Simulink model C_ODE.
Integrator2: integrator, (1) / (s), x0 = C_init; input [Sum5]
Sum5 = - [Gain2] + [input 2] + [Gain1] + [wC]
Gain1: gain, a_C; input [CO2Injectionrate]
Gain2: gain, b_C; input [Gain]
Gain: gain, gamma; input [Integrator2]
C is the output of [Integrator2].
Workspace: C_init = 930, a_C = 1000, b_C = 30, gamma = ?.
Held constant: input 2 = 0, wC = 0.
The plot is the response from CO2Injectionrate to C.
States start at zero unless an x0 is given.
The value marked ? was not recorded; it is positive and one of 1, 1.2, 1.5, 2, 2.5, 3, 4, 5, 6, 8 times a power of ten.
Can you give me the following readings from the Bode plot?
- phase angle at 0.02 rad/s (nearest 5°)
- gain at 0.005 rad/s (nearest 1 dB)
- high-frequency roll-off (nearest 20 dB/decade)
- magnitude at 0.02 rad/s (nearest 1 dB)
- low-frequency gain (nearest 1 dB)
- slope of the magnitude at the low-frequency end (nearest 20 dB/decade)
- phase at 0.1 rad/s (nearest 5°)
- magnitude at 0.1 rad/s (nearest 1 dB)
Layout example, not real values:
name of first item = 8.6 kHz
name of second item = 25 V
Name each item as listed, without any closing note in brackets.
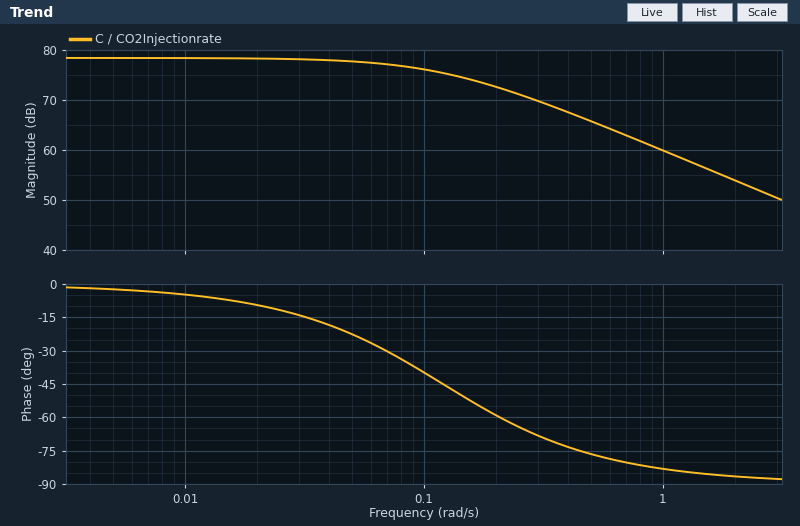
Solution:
phase angle at 0.02 rad/s = -10°
gain at 0.005 rad/s = 78 dB
high-frequency roll-off = -20 dB/decade
magnitude at 0.02 rad/s = 78 dB
low-frequency gain = 78 dB
slope of the magnitude at the low-frequency end = 0 dB/decade
phase at 0.1 rad/s = -40°
magnitude at 0.1 rad/s = 76 dB
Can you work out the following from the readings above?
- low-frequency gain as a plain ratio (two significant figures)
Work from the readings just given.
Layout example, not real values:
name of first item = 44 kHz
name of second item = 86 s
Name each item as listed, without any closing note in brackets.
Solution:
low-frequency gain as a plain ratio = 7900
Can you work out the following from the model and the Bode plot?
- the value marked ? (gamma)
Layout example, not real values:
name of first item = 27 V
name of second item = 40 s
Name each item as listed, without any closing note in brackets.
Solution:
the value marked ? = 0.004
